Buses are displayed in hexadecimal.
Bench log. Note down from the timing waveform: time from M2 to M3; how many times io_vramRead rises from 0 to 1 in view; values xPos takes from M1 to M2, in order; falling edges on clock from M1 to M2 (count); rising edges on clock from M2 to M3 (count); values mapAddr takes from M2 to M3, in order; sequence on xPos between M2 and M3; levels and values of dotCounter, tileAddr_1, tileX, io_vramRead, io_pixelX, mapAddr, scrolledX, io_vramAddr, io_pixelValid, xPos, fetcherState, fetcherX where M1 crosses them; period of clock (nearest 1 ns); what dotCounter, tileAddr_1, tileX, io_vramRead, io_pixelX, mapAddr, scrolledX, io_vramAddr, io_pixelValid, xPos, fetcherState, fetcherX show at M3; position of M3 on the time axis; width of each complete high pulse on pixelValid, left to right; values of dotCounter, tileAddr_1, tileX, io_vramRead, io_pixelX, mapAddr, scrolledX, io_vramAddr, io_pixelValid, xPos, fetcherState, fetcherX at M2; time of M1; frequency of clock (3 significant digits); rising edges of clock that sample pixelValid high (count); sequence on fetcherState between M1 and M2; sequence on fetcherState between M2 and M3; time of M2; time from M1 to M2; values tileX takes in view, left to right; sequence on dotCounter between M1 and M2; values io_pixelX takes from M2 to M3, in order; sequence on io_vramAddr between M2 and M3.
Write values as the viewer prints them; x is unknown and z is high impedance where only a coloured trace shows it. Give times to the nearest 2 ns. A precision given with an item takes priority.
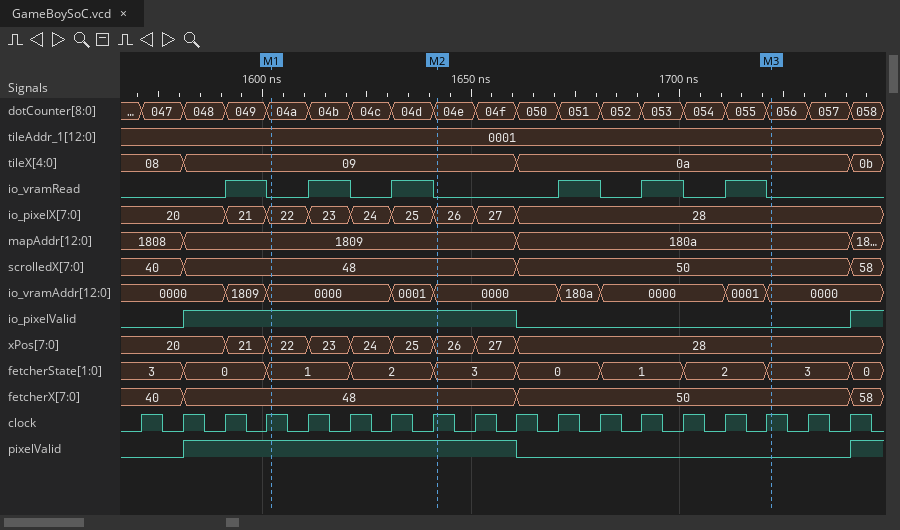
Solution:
80 ns
6
22, 23, 24, 25, 26
4
8
1809, 180a
26, 27, 28
dotCounter=04a, tileAddr_1=0001, tileX=09, io_vramRead=0, io_pixelX=22, mapAddr=1809, scrolledX=48, io_vramAddr=0000, io_pixelValid=1, xPos=22, fetcherState=1, fetcherX=48
10 ns
dotCounter=056, tileAddr_1=0001, tileX=0a, io_vramRead=0, io_pixelX=28, mapAddr=180a, scrolledX=50, io_vramAddr=0000, io_pixelValid=0, xPos=28, fetcherState=3, fetcherX=50
1722 ns
80 ns
dotCounter=04e, tileAddr_1=0001, tileX=09, io_vramRead=0, io_pixelX=26, mapAddr=1809, scrolledX=48, io_vramAddr=0000, io_pixelValid=1, xPos=26, fetcherState=3, fetcherX=48
1602 ns
100 MHz
8
1, 2, 3
3, 0, 1, 2, 3
1642 ns
40 ns
08, 09, 0a, 0b
04a, 04b, 04c, 04d, 04e
26, 27, 28
0000, 180a, 0000, 0001, 0000
